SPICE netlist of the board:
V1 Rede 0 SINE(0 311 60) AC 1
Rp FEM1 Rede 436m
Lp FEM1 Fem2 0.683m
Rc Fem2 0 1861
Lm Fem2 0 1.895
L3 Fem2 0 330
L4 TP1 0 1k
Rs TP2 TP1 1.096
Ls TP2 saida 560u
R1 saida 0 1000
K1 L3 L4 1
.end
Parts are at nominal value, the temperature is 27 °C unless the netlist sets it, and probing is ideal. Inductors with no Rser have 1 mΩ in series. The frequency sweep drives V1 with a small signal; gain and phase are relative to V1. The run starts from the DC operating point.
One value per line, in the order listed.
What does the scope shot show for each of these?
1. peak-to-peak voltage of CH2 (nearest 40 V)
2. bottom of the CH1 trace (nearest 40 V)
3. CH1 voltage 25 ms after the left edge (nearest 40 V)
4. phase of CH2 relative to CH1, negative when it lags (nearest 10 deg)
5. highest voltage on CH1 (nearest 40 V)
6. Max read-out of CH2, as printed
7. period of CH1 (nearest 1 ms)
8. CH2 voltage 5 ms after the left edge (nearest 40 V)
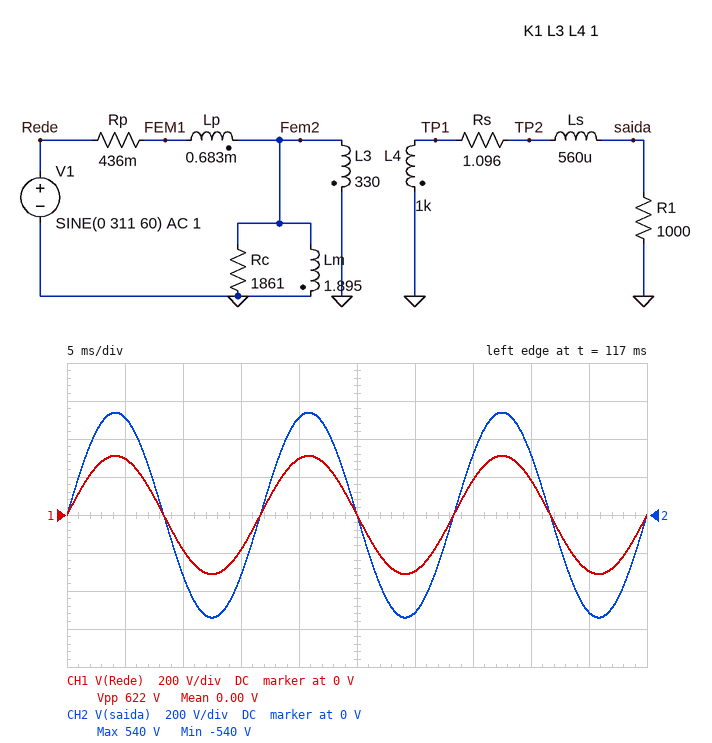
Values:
1.08 kV
-320 V
0 V
0 deg
320 V
540 V
17 ms
520 V
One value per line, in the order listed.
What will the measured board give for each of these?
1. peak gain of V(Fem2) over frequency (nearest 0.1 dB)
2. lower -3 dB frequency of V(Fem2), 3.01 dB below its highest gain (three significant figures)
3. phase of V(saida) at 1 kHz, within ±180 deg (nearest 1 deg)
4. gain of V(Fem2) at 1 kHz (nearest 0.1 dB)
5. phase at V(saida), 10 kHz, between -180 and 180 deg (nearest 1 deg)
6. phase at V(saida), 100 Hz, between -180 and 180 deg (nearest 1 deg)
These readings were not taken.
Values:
0 dB
36.9 mHz
-1 deg
0 dB
-11 deg
0 deg
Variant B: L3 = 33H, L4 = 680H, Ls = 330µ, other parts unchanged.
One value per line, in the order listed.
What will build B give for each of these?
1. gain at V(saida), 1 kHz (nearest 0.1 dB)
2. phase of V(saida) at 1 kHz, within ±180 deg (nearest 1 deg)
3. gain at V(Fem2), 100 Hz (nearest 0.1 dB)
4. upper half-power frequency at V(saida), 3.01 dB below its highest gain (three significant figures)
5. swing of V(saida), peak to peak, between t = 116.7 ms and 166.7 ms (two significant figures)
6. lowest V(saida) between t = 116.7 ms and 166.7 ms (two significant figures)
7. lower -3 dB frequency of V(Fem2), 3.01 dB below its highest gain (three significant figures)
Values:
13.0 dB
-5 deg
-0.1 dB
10.9 kHz
2.8 kV
-1.4 kV
38.5 mHz
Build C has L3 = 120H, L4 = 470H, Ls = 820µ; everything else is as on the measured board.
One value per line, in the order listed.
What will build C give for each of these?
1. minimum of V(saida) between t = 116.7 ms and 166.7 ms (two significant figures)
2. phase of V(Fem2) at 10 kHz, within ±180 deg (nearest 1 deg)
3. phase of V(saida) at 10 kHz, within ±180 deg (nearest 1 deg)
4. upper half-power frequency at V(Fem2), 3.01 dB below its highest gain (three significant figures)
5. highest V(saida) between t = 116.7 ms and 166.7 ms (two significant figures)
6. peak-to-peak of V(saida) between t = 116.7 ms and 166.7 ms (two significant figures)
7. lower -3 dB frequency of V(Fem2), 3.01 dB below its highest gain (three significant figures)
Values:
-610 V
-11 deg
-14 deg
44.3 kHz
610 V
1.2 kV
37.3 mHz
